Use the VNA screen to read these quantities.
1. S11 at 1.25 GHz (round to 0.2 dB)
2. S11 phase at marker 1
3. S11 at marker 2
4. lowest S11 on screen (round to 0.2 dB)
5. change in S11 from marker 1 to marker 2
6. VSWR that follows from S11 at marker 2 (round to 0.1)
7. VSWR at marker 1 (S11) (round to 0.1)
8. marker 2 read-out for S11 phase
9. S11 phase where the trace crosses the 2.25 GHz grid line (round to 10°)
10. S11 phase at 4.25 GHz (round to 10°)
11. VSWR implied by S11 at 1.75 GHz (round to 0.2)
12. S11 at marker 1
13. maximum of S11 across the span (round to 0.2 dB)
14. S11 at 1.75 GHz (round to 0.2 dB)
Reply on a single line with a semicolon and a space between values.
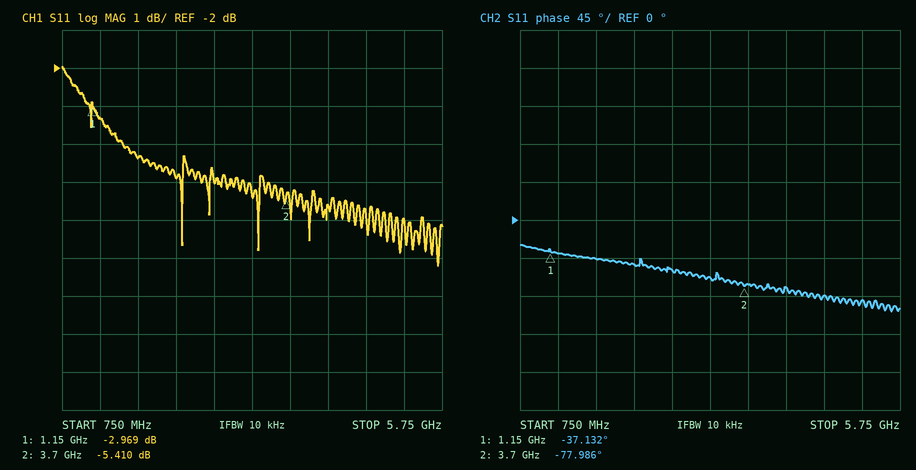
-3.4 dB; -37.132°; -5.410 dB; -7.2 dB; -2.441 dB; 3.3; 5.9; -77.986°; -50°; -80°; 4.0; -2.969 dB; -2.0 dB; -4.4 dB
